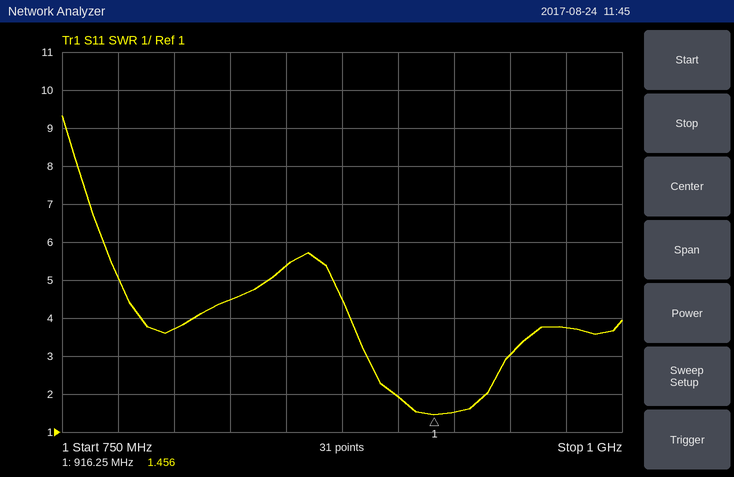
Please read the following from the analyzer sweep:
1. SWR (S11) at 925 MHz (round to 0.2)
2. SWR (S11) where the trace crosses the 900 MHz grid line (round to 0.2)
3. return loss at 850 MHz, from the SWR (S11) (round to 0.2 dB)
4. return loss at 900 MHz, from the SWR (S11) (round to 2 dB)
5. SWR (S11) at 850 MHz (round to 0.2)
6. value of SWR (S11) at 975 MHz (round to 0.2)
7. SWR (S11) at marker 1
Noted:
1.6
2.0
3.2 dB
10 dB
5.4
3.8
1.456
